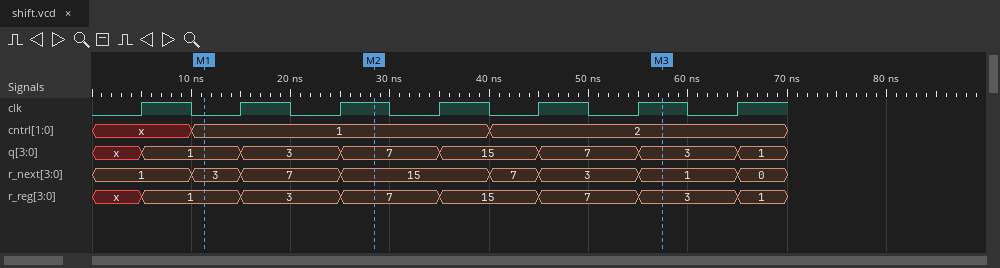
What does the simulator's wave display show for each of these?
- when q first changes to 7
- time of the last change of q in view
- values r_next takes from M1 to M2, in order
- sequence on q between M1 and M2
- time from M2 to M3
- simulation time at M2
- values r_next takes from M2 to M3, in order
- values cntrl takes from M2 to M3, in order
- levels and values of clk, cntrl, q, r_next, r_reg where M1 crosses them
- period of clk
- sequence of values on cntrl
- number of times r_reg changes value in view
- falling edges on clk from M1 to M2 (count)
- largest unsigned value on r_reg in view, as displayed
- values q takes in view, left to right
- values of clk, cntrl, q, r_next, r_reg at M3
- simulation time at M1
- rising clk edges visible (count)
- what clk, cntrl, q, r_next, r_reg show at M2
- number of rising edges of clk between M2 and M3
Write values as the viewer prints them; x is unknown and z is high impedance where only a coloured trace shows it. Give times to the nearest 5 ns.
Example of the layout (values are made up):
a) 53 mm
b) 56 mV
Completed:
a) 25 ns
b) 65 ns
c) 3, 7, 15
d) 1, 3, 7
e) 30 ns
f) 30 ns
g) 15, 7, 3, 1
h) 1, 2
i) clk=0, cntrl=1, q=1, r_next=3, r_reg=1
j) 10 ns
k) x, 1, 2
l) 7
m) 1
n) 15
o) x, 1, 3, 7, 15, 7, 3, 1
p) clk=1, cntrl=2, q=3, r_next=1, r_reg=3
q) 10 ns
r) 7
s) clk=1, cntrl=1, q=7, r_next=15, r_reg=7
t) 3
